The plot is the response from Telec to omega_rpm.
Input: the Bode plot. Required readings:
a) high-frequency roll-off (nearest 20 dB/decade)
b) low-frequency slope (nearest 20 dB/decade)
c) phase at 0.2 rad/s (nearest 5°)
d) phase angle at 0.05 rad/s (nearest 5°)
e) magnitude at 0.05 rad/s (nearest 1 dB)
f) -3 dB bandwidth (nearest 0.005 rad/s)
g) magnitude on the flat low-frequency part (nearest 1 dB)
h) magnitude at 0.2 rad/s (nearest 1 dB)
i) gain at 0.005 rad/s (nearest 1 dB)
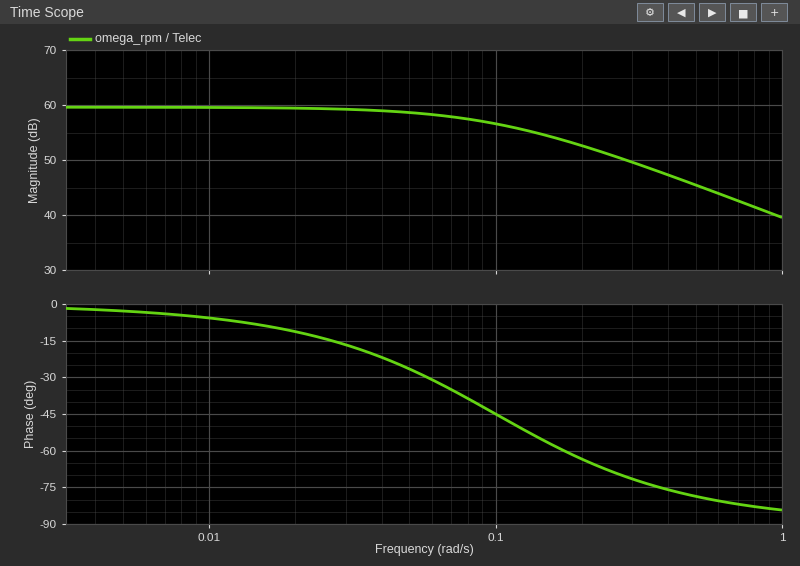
-20 dB/decade
0 dB/decade
-65°
-25°
59 dB
0.100 rad/s
60 dB
53 dB
60 dB
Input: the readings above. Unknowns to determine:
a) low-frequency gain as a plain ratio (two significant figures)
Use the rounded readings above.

1000
